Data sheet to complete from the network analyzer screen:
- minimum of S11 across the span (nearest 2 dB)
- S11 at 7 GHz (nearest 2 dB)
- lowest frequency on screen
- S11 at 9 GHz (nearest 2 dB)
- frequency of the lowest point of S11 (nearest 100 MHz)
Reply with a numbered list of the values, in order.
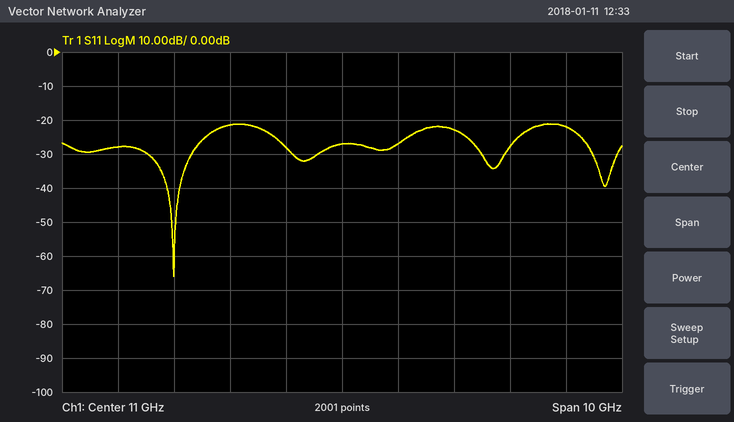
1. -66 dB
2. -28 dB
3. 6 GHz
4. -22 dB
5. 8.0 GHz
